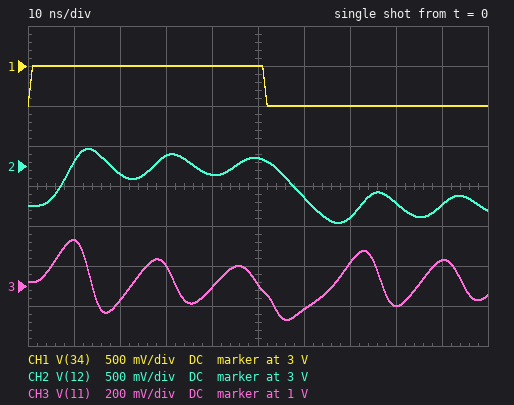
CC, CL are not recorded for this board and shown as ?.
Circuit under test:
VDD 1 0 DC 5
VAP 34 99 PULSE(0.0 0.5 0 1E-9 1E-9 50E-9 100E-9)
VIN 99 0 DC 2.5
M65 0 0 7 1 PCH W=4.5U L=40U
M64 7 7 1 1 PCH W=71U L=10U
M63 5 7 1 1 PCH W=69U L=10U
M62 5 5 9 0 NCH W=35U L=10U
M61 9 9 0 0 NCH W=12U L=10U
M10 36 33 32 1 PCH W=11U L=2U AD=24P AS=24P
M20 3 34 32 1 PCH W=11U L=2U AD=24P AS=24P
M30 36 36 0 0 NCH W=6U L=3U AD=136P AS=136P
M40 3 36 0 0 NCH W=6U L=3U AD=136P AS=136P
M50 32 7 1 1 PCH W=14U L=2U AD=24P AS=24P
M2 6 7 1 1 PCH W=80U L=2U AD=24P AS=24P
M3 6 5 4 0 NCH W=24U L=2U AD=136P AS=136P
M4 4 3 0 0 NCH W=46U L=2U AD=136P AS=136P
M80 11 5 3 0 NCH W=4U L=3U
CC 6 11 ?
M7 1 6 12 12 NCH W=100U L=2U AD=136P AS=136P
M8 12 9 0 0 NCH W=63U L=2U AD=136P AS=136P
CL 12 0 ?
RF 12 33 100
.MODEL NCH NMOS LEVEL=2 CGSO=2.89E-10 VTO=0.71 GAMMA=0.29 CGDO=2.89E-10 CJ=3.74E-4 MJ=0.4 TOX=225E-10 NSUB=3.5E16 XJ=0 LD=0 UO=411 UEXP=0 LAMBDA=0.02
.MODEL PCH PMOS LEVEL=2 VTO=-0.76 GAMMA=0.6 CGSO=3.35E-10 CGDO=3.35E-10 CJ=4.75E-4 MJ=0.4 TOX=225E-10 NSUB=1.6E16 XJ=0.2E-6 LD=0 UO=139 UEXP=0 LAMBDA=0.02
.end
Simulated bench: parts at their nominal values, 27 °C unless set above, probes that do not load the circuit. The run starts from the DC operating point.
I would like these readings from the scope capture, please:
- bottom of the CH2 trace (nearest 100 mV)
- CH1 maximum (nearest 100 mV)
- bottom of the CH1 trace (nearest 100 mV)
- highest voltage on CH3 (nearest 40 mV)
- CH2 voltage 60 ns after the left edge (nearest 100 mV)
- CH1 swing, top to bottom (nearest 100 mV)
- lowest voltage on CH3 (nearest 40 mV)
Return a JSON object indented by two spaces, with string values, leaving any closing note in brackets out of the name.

{
  "bottom of the CH2 trace": "2.3 V",
  "CH1 maximum": "3.0 V",
  "bottom of the CH1 trace": "2.5 V",
  "highest voltage on CH3": "1.24 V",
  "CH2 voltage 60 ns after the left edge": "2.6 V",
  "CH1 swing, top to bottom": "500 mV",
  "lowest voltage on CH3": "840 mV"
}
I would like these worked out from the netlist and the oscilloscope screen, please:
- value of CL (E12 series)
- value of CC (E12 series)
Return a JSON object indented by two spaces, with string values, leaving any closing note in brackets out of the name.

{
  "value of CL": "3.3 pF",
  "value of CC": "120 fF"
}
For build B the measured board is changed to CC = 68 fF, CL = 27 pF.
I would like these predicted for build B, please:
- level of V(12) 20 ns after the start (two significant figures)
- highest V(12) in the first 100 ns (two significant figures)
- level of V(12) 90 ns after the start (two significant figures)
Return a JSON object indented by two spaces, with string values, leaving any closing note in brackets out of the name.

{
  "level of V(12) 20 ns after the start": "3.3 V",
  "highest V(12) in the first 100 ns": "3.4 V",
  "level of V(12) 90 ns after the start": "2.9 V"
}
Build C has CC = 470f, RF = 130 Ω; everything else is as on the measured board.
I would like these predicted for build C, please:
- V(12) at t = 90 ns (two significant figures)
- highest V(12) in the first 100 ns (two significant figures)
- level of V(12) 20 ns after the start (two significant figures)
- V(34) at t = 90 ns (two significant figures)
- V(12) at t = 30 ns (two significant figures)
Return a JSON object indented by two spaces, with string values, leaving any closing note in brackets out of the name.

{
  "V(12) at t = 90 ns": "2.6 V",
  "highest V(12) in the first 100 ns": "3.1 V",
  "level of V(12) 20 ns after the start": "2.7 V",
  "V(34) at t = 90 ns": "2.5 V",
  "V(12) at t = 30 ns": "2.9 V"
}
